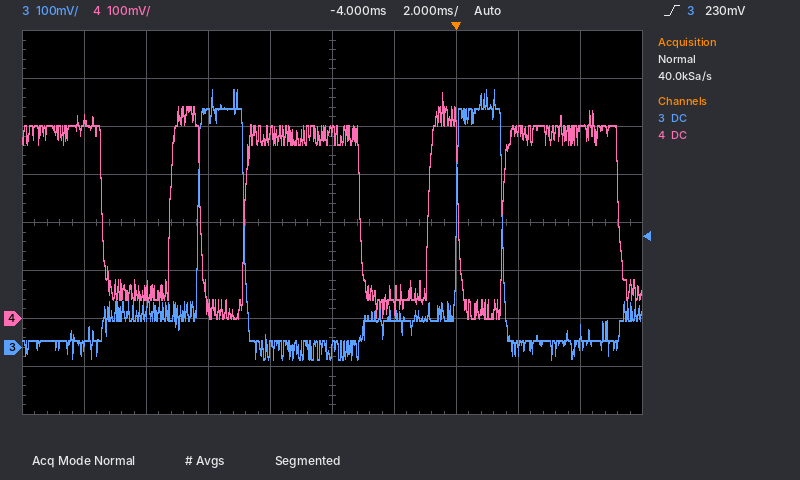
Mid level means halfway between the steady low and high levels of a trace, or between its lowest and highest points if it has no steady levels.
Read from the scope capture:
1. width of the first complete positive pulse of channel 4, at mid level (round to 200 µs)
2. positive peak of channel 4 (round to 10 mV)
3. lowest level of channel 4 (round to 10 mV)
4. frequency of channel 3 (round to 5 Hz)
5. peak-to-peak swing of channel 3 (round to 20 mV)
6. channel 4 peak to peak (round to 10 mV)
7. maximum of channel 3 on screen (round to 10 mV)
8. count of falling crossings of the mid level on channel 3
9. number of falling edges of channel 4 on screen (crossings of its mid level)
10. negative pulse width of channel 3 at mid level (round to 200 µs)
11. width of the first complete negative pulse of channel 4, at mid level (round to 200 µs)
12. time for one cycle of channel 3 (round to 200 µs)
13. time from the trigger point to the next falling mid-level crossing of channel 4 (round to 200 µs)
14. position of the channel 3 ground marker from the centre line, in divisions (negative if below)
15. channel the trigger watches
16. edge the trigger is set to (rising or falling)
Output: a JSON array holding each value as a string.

["1.0 ms", "470 mV", "0 mV", "120 Hz", "560 mV", "470 mV", "540 mV", "2", "5", "6.8 ms", "2.2 ms", "8.4 ms", "5.2 ms", "-2.6 div", "channel 3", "rising"]
